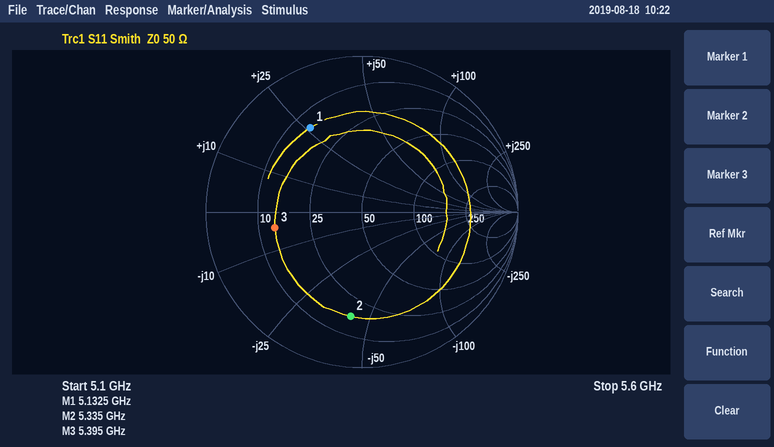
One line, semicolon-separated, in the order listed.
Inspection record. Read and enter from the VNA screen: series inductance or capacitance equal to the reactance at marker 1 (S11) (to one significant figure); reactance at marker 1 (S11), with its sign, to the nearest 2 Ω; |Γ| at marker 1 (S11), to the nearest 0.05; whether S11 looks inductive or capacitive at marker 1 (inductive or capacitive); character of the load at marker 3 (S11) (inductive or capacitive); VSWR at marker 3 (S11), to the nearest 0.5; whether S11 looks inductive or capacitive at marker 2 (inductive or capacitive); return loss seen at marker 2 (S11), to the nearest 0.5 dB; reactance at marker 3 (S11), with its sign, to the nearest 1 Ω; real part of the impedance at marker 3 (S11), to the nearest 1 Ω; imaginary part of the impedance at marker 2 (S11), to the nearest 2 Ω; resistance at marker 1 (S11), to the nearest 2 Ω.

800 pH; +26 Ω; 0.65; inductive; capacitive; 3.5; capacitive; 3.5 dB; -4 Ω; 14 Ω; -42 Ω; 14 Ω
